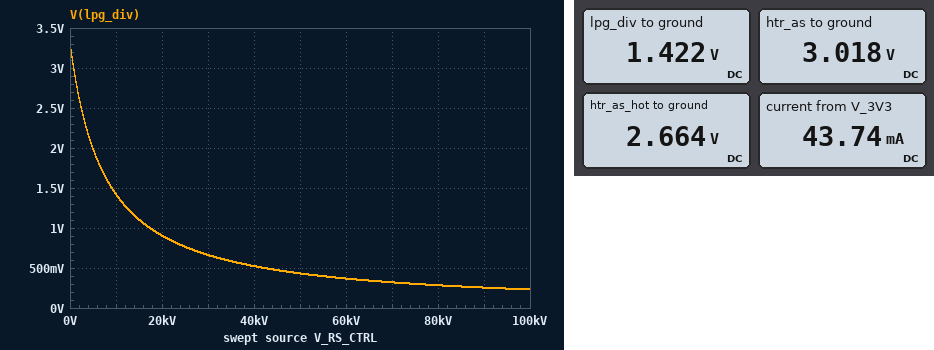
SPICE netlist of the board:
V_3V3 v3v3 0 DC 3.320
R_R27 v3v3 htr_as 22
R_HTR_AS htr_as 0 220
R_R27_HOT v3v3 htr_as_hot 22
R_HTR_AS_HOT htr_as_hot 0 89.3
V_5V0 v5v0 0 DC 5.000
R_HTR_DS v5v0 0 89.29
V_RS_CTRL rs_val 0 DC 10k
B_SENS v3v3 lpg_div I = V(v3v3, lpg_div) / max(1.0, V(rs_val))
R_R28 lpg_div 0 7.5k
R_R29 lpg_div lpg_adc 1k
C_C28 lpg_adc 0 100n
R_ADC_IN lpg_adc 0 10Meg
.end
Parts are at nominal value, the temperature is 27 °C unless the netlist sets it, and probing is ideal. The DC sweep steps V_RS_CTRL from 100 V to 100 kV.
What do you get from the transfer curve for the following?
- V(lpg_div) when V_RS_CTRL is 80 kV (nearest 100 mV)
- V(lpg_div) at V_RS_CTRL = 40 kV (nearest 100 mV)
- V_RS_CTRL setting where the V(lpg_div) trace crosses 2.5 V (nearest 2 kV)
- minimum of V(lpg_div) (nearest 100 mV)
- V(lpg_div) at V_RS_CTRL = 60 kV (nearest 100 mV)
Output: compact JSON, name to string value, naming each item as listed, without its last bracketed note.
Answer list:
{"V(lpg_div) when V_RS_CTRL is 80 kV": "300 mV", "V(lpg_div) at V_RS_CTRL = 40 kV": "500 mV", "V_RS_CTRL setting where the V(lpg_div) trace crosses 2.5 V": "2 kV", "minimum of V(lpg_div)": "200 mV", "V(lpg_div) at V_RS_CTRL = 60 kV": "400 mV"}
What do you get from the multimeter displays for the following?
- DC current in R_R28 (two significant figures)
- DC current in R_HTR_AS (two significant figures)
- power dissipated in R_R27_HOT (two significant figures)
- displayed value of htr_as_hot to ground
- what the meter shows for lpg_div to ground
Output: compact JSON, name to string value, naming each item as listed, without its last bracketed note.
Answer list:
{"DC current in R_R28": "190 µA", "DC current in R_HTR_AS": "14 mA", "power dissipated in R_R27_HOT": "20 mW", "displayed value of htr_as_hot to ground": "2.664 V", "what the meter shows for lpg_div to ground": "1.422 V"}
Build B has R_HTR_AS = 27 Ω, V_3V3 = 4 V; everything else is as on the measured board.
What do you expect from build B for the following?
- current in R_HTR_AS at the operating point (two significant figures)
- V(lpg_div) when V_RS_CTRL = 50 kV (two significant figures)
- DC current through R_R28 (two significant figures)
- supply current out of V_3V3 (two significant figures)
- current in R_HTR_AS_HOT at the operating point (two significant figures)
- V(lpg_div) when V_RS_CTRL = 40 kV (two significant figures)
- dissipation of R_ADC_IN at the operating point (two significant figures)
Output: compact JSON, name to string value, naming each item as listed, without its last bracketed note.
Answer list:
{"current in R_HTR_AS at the operating point": "82 mA", "V(lpg_div) when V_RS_CTRL = 50 kV": "520 mV", "DC current through R_R28": "230 µA", "supply current out of V_3V3": "120 mA", "current in R_HTR_AS_HOT at the operating point": "36 mA", "V(lpg_div) when V_RS_CTRL = 40 kV": "630 mV", "dissipation of R_ADC_IN at the operating point": "290 nW"}
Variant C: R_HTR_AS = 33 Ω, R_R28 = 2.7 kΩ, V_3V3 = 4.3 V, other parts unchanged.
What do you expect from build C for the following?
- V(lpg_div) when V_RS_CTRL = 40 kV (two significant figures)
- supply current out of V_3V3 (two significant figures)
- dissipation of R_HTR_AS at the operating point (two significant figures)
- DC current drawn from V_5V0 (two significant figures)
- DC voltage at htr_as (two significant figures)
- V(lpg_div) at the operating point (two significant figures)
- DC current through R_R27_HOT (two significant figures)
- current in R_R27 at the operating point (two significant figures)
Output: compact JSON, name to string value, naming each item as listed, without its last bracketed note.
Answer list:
{"V(lpg_div) when V_RS_CTRL = 40 kV": "270 mV", "supply current out of V_3V3": "120 mA", "dissipation of R_HTR_AS at the operating point": "200 mW", "DC current drawn from V_5V0": "56 mA", "DC voltage at htr_as": "2.6 V", "V(lpg_div) at the operating point": "910 mV", "DC current through R_R27_HOT": "39 mA", "current in R_R27 at the operating point": "78 mA"}
